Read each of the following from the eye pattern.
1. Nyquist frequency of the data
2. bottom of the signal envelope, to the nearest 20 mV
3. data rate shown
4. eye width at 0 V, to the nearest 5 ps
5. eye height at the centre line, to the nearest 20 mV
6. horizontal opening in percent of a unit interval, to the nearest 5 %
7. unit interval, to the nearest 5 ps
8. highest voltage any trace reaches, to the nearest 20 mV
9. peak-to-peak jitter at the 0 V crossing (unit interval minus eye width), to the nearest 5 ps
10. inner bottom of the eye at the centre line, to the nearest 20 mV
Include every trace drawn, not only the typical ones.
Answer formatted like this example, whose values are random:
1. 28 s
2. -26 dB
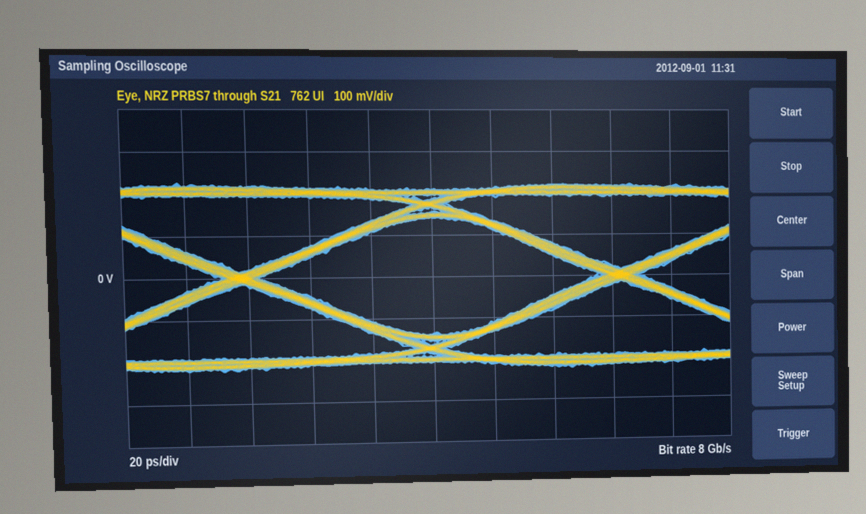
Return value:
1. 4 GHz
2. -220 mV
3. 8 Gb/s
4. 110 ps
5. 280 mV
6. 90 %
7. 125 ps
8. 220 mV
9. 15 ps
10. -140 mV
